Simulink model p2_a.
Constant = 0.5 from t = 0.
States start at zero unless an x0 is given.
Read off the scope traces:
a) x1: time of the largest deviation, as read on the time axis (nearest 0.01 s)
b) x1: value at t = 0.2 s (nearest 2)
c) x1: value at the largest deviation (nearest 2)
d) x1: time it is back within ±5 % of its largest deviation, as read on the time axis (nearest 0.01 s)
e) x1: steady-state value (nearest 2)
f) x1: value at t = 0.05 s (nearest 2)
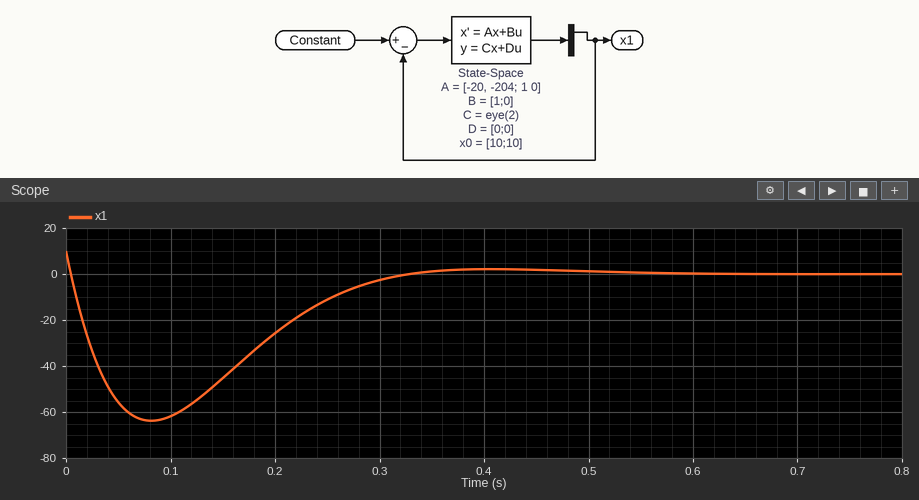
0.08 s
-26
-64
0.29 s
0
-56
